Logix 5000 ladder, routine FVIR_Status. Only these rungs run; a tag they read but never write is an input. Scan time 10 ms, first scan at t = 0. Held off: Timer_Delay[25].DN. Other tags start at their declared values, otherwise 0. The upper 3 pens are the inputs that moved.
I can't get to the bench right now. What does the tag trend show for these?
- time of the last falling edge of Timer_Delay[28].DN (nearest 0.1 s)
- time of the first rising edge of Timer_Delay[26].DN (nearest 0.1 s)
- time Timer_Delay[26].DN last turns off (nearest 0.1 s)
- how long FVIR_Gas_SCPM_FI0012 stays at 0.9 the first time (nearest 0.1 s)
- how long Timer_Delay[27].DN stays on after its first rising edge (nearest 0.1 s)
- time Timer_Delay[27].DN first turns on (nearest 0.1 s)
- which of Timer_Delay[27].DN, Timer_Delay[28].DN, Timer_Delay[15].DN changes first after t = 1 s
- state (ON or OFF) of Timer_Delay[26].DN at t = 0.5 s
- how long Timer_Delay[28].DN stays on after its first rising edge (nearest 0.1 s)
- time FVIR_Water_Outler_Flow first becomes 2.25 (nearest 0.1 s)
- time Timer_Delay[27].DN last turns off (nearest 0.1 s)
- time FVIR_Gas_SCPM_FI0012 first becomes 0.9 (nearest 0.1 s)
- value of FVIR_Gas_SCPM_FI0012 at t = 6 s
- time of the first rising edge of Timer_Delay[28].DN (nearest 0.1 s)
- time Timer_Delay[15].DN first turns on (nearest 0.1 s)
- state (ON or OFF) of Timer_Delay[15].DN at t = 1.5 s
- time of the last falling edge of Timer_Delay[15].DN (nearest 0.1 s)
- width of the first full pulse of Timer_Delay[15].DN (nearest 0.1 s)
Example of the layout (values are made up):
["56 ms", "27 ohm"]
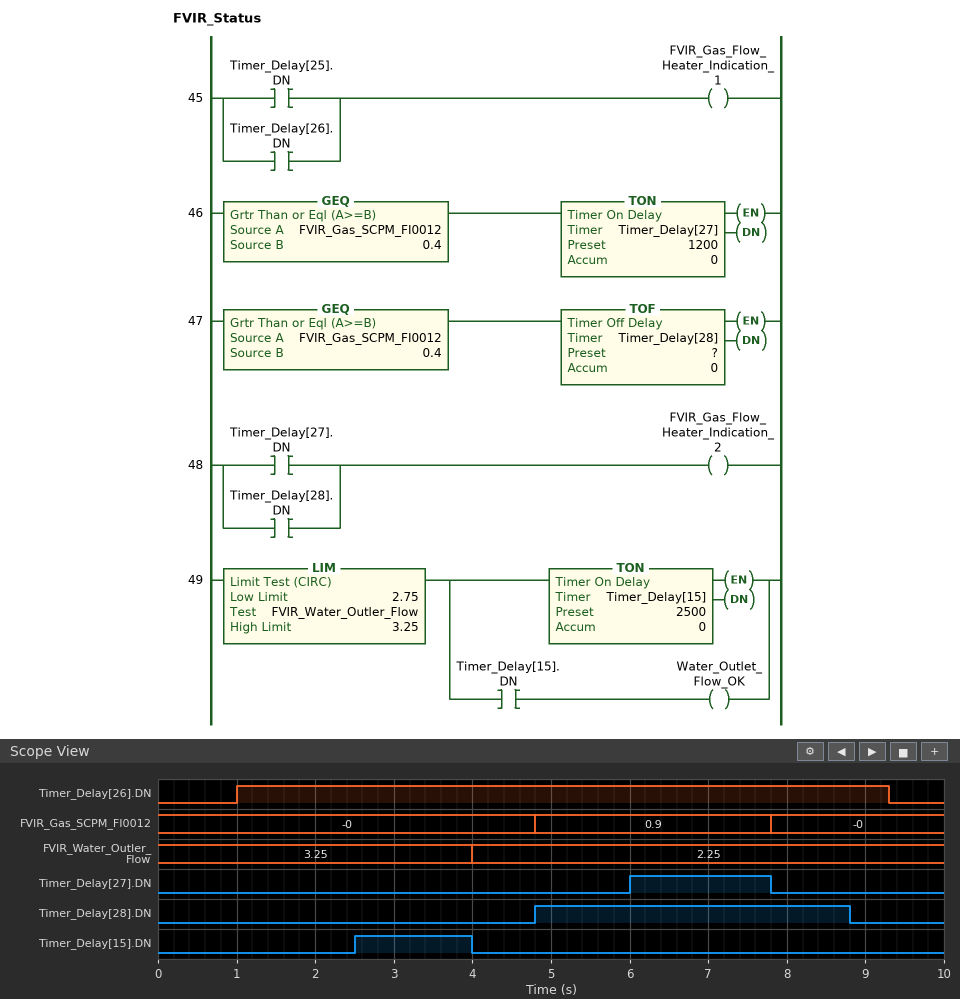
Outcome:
["8.8 s", "1.0 s", "9.3 s", "3.0 s", "1.8 s", "6.0 s", "Timer_Delay[15].DN", "OFF", "4.0 s", "4.0 s", "7.8 s", "4.8 s", "0.9", "4.8 s", "2.5 s", "OFF", "4.0 s", "1.5 s"]
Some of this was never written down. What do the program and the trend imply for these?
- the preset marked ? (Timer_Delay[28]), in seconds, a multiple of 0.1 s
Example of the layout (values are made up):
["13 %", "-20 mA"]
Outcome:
["1.0 s"]
